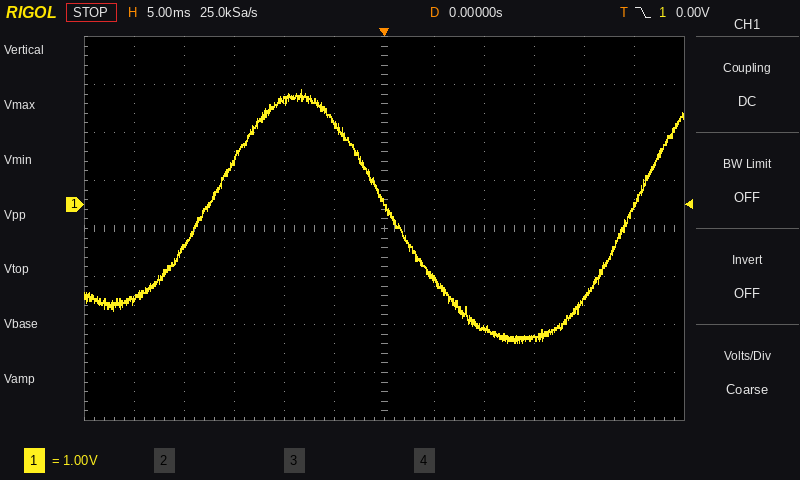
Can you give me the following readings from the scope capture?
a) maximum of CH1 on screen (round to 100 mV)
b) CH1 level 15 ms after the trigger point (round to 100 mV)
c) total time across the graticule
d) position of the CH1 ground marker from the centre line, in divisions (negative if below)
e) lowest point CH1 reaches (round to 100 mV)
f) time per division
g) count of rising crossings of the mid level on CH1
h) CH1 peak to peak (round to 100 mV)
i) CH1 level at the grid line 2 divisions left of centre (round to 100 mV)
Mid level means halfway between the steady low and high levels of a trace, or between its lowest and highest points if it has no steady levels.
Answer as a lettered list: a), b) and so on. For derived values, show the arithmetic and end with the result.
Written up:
a) 2.4 V
b) -2.8 V
c) 60 ms
d) +0.5 div
e) -2.9 V
f) 5 ms
g) 2
h) 2.4 V − (-2.9 V) = 5.3 V
i) 2.2 V
